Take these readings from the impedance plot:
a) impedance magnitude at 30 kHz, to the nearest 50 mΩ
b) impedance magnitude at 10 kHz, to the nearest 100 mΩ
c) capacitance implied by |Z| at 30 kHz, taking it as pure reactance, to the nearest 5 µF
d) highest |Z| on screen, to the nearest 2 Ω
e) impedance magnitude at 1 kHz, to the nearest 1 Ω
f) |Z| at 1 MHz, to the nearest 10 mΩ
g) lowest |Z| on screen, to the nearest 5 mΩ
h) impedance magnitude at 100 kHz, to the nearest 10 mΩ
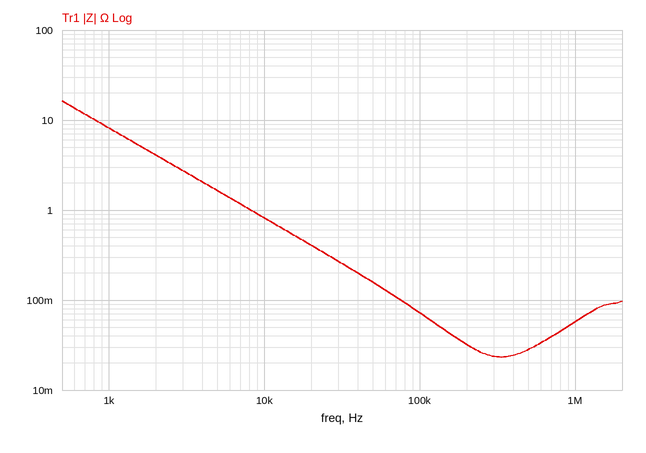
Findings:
250 mΩ
800 mΩ
20 µF
16 Ω
8 Ω
60 mΩ
25 mΩ
70 mΩ
